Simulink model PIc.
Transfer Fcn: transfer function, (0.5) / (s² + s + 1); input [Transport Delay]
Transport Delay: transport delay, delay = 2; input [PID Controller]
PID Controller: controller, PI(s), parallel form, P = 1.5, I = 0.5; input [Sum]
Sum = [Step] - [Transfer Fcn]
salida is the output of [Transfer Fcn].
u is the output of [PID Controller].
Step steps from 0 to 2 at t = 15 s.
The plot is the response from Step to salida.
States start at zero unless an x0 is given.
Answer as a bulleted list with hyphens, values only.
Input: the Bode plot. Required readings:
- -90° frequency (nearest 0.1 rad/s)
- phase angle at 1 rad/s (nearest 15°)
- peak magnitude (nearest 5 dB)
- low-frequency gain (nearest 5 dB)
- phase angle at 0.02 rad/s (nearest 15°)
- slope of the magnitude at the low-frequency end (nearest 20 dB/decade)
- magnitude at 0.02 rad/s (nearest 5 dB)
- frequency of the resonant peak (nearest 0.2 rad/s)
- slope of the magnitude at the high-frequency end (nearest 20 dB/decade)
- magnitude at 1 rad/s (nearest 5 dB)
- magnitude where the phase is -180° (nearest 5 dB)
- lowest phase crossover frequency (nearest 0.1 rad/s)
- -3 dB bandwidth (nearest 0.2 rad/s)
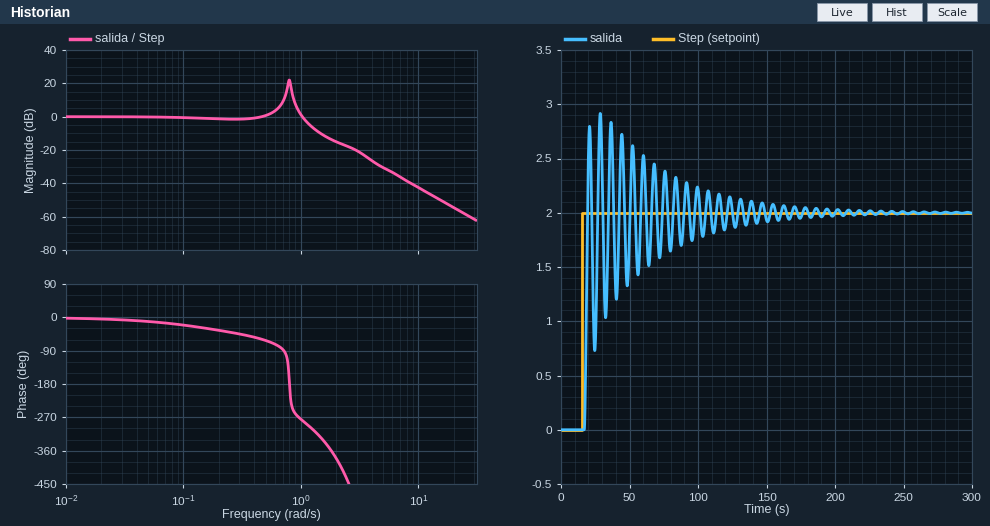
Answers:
- 0.7 rad/s
- -270°
- 20 dB
- 0 dB
- 0°
- 0 dB/decade
- 0 dB
- 0.8 rad/s
- -40 dB/decade
- 0 dB
- 20 dB
- 0.8 rad/s
- 1.2 rad/s
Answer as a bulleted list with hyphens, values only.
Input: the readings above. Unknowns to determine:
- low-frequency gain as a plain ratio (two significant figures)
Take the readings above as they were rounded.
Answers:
- 1.0
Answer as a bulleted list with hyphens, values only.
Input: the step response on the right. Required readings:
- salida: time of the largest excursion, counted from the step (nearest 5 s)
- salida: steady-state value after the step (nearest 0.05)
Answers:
- 15 s
- 2.00
